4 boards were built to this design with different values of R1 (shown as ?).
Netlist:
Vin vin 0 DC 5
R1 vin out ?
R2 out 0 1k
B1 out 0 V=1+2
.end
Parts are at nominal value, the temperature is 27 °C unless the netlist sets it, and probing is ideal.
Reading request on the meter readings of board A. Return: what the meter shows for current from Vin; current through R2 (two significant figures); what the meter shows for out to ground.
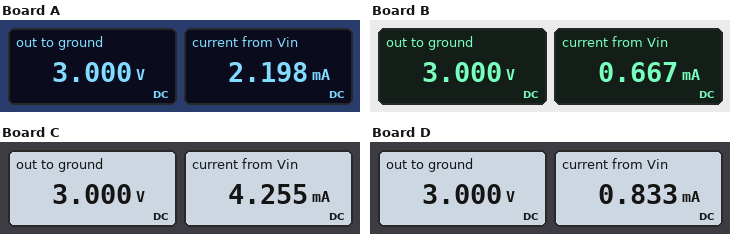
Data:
2.198 mA
3.0 mA
3.000 V
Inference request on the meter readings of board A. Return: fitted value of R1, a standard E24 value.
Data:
910 Ω
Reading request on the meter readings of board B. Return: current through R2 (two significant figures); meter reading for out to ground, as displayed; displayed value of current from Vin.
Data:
3.0 mA
3.000 V
0.667 mA
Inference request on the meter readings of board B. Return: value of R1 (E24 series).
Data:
3 kΩ
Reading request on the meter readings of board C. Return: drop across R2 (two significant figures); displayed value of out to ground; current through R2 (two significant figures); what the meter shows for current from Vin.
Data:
3.0 V
3.000 V
3.0 mA
4.255 mA
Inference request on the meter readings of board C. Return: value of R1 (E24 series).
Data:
470 Ω
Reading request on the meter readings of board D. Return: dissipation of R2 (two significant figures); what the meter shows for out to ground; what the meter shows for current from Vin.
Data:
9.0 mW
3.000 V
0.833 mA
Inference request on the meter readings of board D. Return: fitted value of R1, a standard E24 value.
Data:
2.4 kΩ
